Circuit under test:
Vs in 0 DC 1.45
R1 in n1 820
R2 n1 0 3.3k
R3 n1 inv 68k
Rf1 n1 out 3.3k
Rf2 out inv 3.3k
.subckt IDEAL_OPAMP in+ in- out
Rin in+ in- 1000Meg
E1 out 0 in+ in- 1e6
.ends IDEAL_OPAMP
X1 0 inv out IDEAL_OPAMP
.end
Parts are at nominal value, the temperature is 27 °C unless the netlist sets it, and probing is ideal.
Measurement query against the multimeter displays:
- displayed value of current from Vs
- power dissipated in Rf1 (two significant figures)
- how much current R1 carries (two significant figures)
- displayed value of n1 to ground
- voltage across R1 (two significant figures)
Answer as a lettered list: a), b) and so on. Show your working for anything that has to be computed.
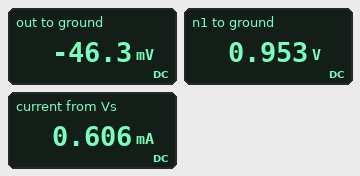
a) 0.606 mA
b) (953 mV - (-46.3 mV))^2 / 3.3 kΩ = 300 µW
c) (1.45 V - 953 mV) / 820 Ω = 610 µA
d) 0.953 V
e) 1.45 V - 953 mV = 500 mV
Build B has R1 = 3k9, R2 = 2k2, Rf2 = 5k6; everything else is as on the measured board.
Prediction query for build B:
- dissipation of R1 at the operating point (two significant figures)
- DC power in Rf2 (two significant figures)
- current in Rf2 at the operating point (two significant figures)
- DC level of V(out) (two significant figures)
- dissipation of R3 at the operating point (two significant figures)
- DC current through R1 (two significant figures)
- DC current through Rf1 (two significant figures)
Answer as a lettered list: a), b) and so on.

a) 310 µW
b) 150 nW
c) 5.2 µA
d) -29 mV
e) 1.8 µW
f) 280 µA
g) 120 µA
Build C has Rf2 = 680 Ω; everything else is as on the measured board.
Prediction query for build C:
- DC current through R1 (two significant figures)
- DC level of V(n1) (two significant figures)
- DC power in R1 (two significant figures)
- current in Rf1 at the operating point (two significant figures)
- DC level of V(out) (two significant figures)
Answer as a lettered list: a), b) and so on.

a) 600 µA
b) 960 mV
c) 290 µW
d) 290 µA
e) -9.6 mV
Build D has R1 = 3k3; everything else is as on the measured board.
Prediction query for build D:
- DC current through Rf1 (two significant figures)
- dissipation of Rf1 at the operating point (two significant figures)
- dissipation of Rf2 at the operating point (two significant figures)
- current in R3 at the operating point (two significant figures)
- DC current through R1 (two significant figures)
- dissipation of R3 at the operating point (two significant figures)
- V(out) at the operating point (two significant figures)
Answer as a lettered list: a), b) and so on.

a) 150 µA
b) 73 µW
c) 160 nW
d) 6.9 µA
e) 300 µA
f) 3.2 µW
g) -23 mV
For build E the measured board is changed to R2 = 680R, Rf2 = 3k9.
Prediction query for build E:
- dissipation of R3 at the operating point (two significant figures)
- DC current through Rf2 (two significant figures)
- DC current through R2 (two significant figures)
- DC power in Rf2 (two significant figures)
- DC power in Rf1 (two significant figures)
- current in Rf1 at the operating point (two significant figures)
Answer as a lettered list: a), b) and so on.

a) 5.0 µW
b) 8.6 µA
c) 860 µA
d) 290 nW
e) 120 µW
f) 190 µA
